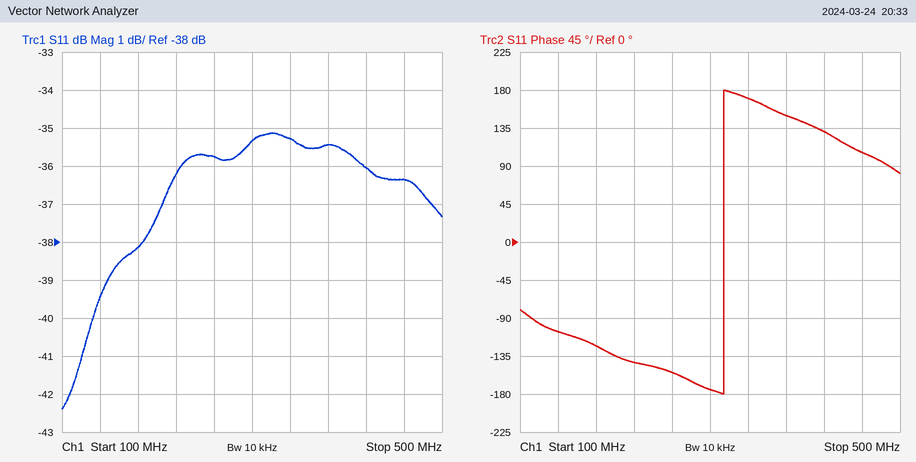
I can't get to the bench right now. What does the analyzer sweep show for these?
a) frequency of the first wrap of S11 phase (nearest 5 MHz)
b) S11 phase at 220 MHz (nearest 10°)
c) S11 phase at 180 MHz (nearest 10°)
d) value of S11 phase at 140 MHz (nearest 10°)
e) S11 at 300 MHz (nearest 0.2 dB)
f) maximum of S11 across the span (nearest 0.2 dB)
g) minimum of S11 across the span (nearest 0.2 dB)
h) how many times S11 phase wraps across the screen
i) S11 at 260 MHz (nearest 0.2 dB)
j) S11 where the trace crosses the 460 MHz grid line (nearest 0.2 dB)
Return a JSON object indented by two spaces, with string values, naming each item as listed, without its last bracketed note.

{
  "frequency of the first wrap of S11 phase": "315 MHz",
  "S11 phase at 220 MHz": "-140°",
  "S11 phase at 180 MHz": "-120°",
  "value of S11 phase at 140 MHz": "-110°",
  "S11 at 300 MHz": "-35.4 dB",
  "maximum of S11 across the span": "-35.2 dB",
  "minimum of S11 across the span": "-42.4 dB",
  "how many times S11 phase wraps across the screen": "1",
  "S11 at 260 MHz": "-35.8 dB",
  "S11 where the trace crosses the 460 MHz grid line": "-36.4 dB"
}
